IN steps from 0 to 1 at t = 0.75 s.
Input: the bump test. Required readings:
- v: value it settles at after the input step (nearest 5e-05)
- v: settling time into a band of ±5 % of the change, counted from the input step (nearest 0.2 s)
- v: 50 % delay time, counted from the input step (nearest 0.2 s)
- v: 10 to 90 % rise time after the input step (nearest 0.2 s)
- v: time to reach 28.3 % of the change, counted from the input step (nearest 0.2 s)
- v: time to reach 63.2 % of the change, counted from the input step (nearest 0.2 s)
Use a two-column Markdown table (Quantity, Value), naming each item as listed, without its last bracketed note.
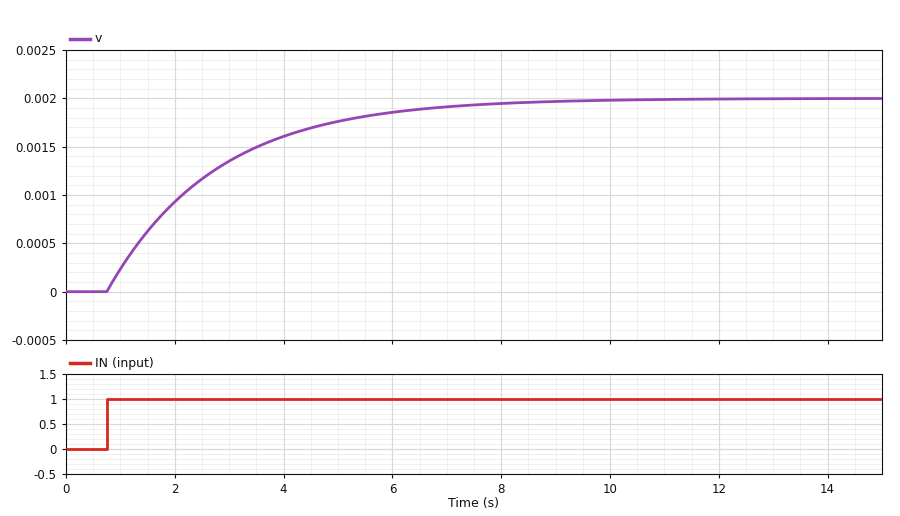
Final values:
| Quantity | Value |
|---|---|
| v: value it settles at after the input step | 0.00200 |
| v: settling time into a band of ±5 % of the change, counted from the input step | 6.0 s |
| v: 50 % delay time, counted from the input step | 1.4 s |
| v: 10 to 90 % rise time after the input step | 4.4 s |
| v: time to reach 28.3 % of the change, counted from the input step | 0.6 s |
| v: time to reach 63.2 % of the change, counted from the input step | 2.0 s |
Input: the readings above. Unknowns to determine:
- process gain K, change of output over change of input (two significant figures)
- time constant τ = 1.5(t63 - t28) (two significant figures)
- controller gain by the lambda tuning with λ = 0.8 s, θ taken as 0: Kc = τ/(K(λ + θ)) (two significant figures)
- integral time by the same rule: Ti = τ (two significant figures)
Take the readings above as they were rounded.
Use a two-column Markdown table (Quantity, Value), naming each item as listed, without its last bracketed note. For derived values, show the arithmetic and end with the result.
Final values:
| Quantity | Value |
|---|---|
| process gain K, change of output over change of input | (0.002 - 0) / 1 = 0.0020 |
| time constant τ = 1.5(t63 - t28) | 1.5 × (2 - 0.6) = 2.1 s |
| controller gain by the lambda tuning with λ = 0.8 s, θ taken as 0: Kc = τ/(K(λ + θ)) | 2.1 / (0.002 × (0.8 + 0)) = 1300 |
| integral time by the same rule: Ti = τ | 2.1 s |
